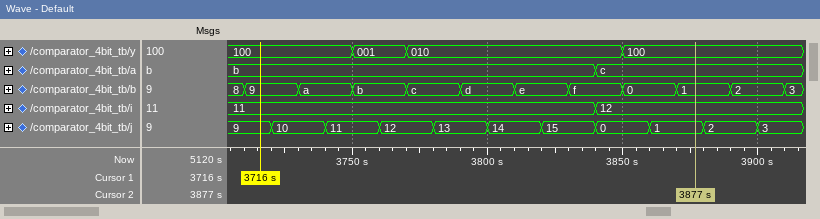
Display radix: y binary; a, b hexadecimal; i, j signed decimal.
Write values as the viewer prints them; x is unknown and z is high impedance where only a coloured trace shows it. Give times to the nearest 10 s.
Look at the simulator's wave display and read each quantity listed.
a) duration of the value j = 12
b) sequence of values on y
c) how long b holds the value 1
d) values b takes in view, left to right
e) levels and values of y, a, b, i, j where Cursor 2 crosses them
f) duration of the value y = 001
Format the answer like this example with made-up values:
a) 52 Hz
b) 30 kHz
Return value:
a) 20 s
b) 100, 001, 010, 100
c) 20 s
d) 8, 9, a, b, c, d, e, f, 0, 1, 2, 3
e) y=100, a=c, b=1, i=12, j=1
f) 20 s
